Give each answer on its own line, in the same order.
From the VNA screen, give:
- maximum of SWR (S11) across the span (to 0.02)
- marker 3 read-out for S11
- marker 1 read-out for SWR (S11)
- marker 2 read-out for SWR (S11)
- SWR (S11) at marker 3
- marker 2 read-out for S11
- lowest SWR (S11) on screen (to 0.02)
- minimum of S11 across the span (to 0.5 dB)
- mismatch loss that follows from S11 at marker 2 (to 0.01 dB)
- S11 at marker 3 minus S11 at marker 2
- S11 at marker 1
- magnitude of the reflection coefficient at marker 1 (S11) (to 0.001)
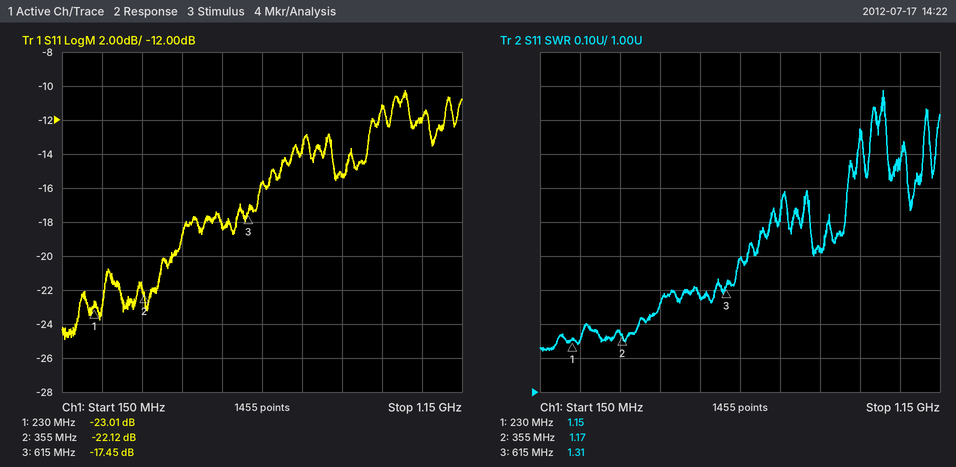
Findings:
1.88
-17.45 dB
1.15
1.17
1.31
-22.12 dB
1.12
-25.0 dB
0.03 dB
4.67 dB
-23.01 dB
0.071
